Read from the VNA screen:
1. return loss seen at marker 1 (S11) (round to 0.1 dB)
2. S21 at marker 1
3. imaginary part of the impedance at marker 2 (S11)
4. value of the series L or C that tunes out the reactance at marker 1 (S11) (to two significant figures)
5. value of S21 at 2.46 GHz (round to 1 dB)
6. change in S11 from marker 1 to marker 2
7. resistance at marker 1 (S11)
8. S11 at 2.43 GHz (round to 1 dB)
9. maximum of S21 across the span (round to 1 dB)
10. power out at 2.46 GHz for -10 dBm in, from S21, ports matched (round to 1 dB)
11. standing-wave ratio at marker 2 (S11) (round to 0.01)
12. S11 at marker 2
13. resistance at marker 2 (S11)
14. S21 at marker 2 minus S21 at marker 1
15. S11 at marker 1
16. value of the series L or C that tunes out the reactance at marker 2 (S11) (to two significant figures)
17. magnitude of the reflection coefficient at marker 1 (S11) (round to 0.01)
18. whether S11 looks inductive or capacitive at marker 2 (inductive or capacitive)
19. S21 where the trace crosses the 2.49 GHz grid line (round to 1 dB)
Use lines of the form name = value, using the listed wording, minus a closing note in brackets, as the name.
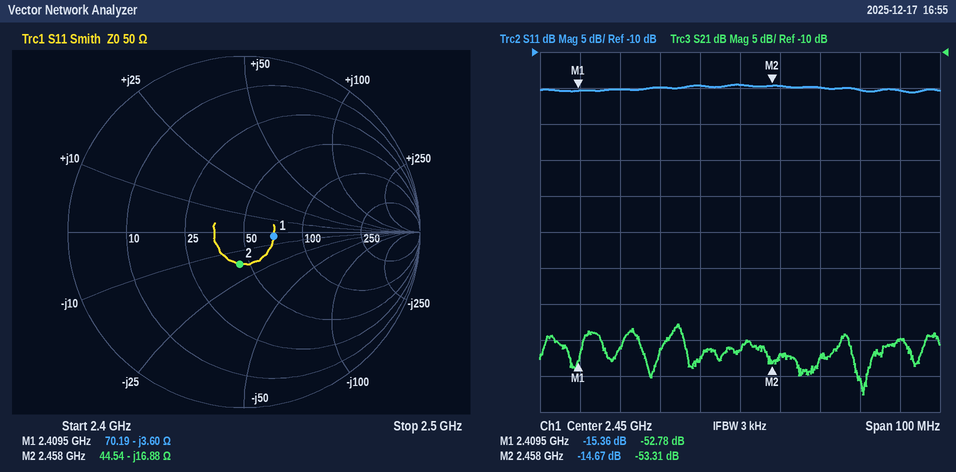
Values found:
return loss seen at marker 1 (S11) = 15.4 dB
S21 at marker 1 = -52.78 dB
imaginary part of the impedance at marker 2 = -16.88 Ω
value of the series L or C that tunes out the reactance at marker 1 (S11) = 240 pH
value of S21 at 2.46 GHz = -52 dB
change in S11 from marker 1 to marker 2 = 0.69 dB
resistance at marker 1 = 70.19 Ω
S11 at 2.43 GHz = -15 dB
maximum of S21 across the span = -48 dB
power out at 2.46 GHz for -10 dBm in, from S21, ports matched = -62 dBm
standing-wave ratio at marker 2 (S11) = 1.45
S11 at marker 2 = -14.67 dB
resistance at marker 2 = 44.54 Ω
S21 at marker 2 minus S21 at marker 1 = -0.53 dB
S11 at marker 1 = -15.36 dB
value of the series L or C that tunes out the reactance at marker 2 (S11) = 1.1 nH
magnitude of the reflection coefficient at marker 1 (S11) = 0.17
whether S11 looks inductive or capacitive at marker 2 = capacitive
S21 where the trace crosses the 2.49 GHz grid line = -50 dB
